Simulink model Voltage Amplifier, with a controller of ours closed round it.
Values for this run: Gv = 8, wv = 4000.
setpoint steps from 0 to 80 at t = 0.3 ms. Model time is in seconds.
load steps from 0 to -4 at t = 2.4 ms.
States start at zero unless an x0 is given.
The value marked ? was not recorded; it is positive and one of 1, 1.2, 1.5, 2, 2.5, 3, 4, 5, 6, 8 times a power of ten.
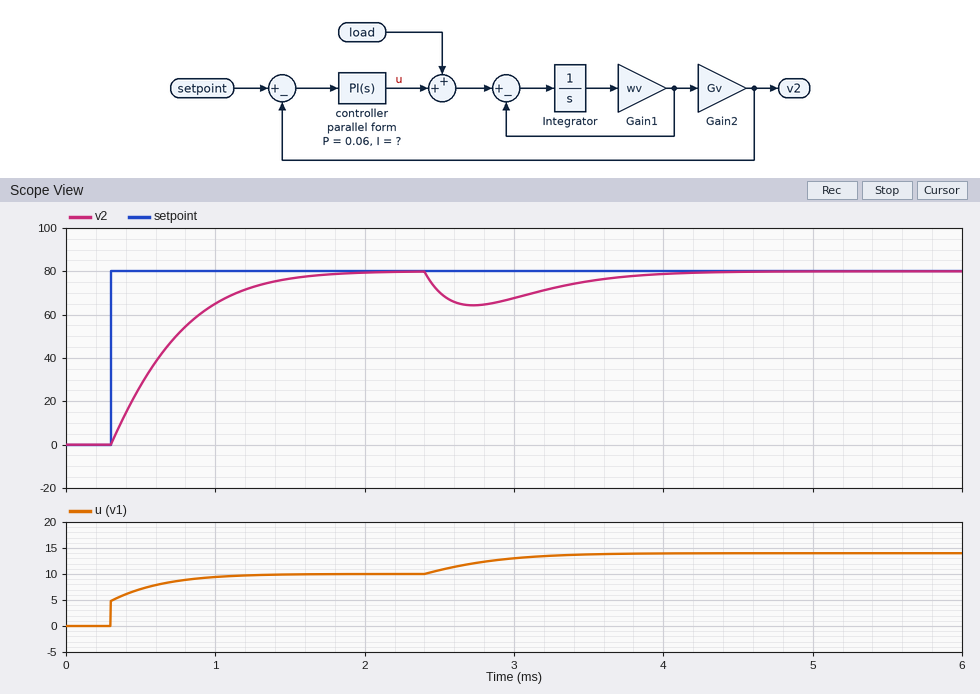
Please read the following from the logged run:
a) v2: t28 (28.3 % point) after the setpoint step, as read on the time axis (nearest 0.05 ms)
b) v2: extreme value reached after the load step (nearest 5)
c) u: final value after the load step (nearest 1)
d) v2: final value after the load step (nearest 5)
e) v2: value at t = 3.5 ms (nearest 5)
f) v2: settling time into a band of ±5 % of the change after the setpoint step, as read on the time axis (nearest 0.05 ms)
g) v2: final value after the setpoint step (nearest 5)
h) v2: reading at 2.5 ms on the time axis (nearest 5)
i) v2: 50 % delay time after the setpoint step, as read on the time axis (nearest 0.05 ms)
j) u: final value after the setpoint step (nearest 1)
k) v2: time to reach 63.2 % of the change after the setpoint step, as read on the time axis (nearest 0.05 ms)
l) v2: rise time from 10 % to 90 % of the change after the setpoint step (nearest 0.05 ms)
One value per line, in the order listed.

0.45 ms
65
14
80
75
1.45 ms
80
70
0.60 ms
10
0.75 ms
0.85 ms
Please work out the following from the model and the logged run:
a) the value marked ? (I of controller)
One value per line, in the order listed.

300
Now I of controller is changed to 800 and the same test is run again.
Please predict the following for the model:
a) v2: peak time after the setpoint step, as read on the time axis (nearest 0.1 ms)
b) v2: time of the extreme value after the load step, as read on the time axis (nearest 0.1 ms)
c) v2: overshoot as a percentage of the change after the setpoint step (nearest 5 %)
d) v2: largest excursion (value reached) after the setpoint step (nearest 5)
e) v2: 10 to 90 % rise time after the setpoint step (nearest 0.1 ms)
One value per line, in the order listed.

1.0 ms
2.6 ms
10 %
90
0.3 ms
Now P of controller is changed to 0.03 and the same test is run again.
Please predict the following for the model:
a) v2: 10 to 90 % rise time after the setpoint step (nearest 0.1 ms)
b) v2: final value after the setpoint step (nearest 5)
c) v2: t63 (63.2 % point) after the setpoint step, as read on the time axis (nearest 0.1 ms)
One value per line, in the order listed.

0.8 ms
80
0.8 ms
